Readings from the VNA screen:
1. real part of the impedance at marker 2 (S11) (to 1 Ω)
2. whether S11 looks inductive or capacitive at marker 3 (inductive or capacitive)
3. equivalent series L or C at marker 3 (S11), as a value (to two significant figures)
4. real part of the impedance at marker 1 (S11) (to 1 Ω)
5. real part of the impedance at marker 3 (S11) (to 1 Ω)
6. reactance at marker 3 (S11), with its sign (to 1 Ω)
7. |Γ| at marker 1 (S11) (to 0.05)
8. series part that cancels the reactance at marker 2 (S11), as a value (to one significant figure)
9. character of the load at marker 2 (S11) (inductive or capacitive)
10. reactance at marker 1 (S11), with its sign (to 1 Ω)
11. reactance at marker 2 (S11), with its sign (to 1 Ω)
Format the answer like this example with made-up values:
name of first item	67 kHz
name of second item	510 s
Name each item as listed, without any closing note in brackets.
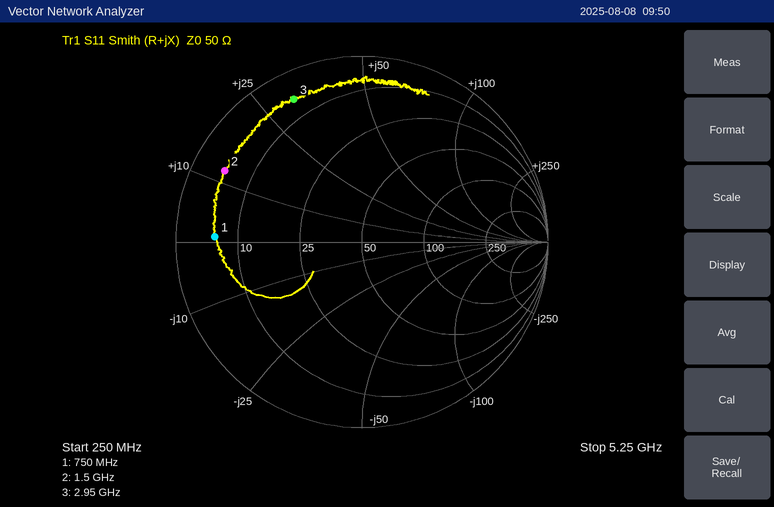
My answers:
real part of the impedance at marker 2 (S11)	5 Ω
whether S11 looks inductive or capacitive at marker 3	inductive
equivalent series L or C at marker 3 (S11), as a value	1.7 nH
real part of the impedance at marker 1 (S11)	6 Ω
real part of the impedance at marker 3 (S11)	6 Ω
reactance at marker 3 (S11), with its sign	+31 Ω
|Γ| at marker 1 (S11)	0.80
series part that cancels the reactance at marker 2 (S11), as a value	9 pF
character of the load at marker 2 (S11)	inductive
reactance at marker 1 (S11), with its sign	+1 Ω
reactance at marker 2 (S11), with its sign	+12 Ω
